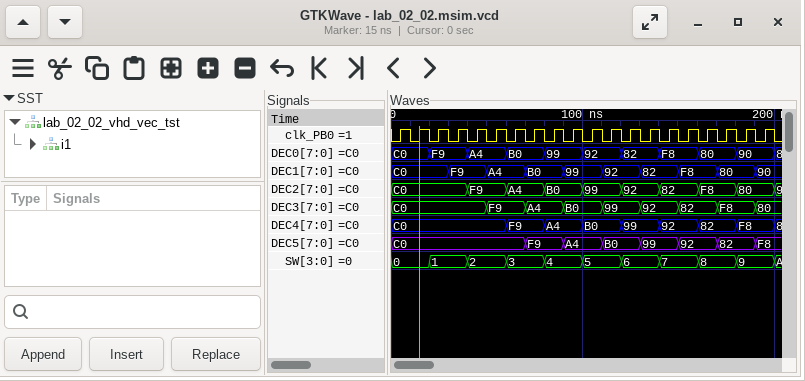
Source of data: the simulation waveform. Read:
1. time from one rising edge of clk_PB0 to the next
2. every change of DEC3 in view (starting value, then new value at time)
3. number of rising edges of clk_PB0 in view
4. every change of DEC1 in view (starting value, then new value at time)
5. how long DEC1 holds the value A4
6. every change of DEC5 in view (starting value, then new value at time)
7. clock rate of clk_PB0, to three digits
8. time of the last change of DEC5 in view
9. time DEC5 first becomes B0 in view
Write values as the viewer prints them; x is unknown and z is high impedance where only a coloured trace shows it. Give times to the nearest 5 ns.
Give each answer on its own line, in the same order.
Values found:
10 ns
C0, F9 at 50 ns, A4 at 70 ns, B0 at 90 ns, 99 at 110 ns, 92 at 130 ns, 82 at 150 ns, F8 at 170 ns, 80 at 190 ns
20
C0, F9 at 30 ns, A4 at 50 ns, B0 at 70 ns, 99 at 90 ns, 92 at 110 ns, 82 at 130 ns, F8 at 150 ns, 80 at 170 ns, 90 at 190 ns
20 ns
C0, F9 at 70 ns, A4 at 90 ns, B0 at 110 ns, 99 at 130 ns, 92 at 150 ns, 82 at 170 ns, F8 at 190 ns
100 MHz
190 ns
110 ns
